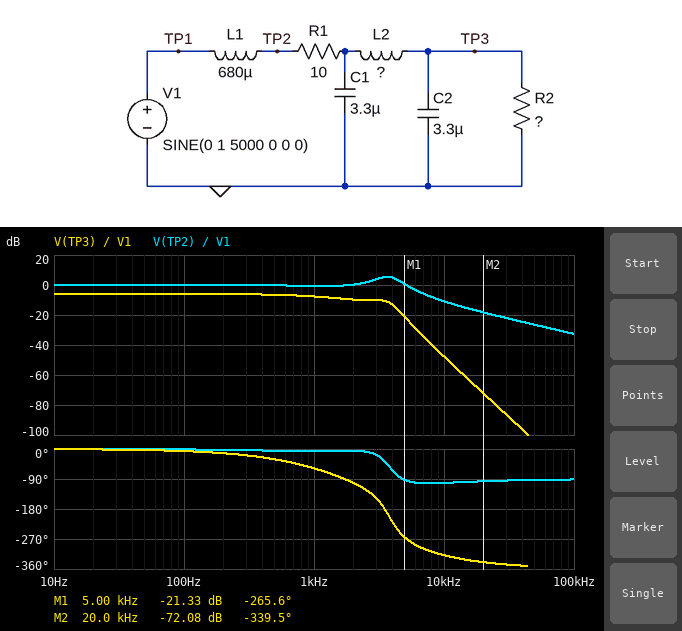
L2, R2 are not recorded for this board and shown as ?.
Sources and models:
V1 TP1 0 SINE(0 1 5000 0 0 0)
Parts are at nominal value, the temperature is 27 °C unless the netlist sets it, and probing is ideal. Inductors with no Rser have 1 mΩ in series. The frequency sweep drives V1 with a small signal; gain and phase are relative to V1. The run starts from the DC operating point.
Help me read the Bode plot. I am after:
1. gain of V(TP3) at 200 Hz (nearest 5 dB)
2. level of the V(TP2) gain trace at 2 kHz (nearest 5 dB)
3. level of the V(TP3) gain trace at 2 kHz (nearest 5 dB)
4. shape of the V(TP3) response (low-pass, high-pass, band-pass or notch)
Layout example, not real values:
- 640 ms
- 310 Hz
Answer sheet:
- -5 dB
- 0 dB
- -10 dB
- low-pass
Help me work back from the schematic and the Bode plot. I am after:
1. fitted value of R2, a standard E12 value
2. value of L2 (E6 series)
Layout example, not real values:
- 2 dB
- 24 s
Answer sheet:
- 10 Ω
- 2.2 mH
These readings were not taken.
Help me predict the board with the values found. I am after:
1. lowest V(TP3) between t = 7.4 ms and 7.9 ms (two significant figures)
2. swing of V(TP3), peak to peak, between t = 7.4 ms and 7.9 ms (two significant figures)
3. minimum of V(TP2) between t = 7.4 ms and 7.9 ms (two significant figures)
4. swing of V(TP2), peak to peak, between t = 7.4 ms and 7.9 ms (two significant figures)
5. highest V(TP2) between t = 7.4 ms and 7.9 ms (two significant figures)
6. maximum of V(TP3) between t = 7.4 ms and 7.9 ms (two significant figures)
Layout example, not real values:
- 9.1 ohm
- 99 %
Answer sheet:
- -86 mV
- 170 mV
- -1.1 V
- 2.1 V
- 1.1 V
- 86 mV
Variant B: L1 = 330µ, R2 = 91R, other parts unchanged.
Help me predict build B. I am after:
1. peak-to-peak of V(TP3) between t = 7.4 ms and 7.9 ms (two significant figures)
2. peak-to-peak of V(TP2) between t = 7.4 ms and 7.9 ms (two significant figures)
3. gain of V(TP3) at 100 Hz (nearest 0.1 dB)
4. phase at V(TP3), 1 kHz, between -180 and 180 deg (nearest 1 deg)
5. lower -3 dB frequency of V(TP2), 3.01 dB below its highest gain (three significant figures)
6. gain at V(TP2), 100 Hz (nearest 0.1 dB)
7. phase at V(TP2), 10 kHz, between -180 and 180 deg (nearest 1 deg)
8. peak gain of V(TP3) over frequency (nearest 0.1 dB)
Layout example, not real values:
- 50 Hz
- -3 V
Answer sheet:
- 370 mV
- 3.0 V
- -0.9 dB
- -36 deg
- 2.85 kHz
- 0 dB
- -84 deg
- 3.4 dB
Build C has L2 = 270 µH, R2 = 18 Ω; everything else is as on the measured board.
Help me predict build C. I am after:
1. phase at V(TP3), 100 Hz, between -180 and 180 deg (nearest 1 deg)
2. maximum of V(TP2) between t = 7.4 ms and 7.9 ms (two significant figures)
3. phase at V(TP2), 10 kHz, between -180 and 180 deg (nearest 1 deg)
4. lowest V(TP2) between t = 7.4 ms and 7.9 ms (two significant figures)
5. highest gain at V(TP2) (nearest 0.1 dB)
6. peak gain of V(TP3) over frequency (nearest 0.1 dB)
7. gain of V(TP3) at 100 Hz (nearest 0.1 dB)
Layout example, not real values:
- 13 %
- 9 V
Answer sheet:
- -3 deg
- 570 mV
- -110 deg
- -570 mV
- 0.7 dB
- -3.5 dB
- -3.8 dB
